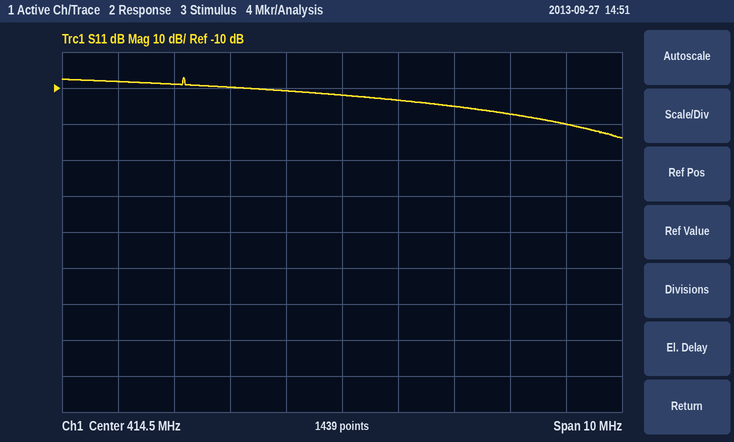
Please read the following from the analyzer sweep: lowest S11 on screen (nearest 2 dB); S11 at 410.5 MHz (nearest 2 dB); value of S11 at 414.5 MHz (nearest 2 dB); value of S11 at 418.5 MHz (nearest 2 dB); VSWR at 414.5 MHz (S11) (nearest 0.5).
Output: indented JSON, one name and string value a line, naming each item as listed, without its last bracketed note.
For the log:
{
  "lowest S11 on screen": "-24 dB",
  "S11 at 410.5 MHz": "-8 dB",
  "value of S11 at 414.5 MHz": "-12 dB",
  "value of S11 at 418.5 MHz": "-20 dB",
  "VSWR at 414.5 MHz (S11)": "1.5"
}
